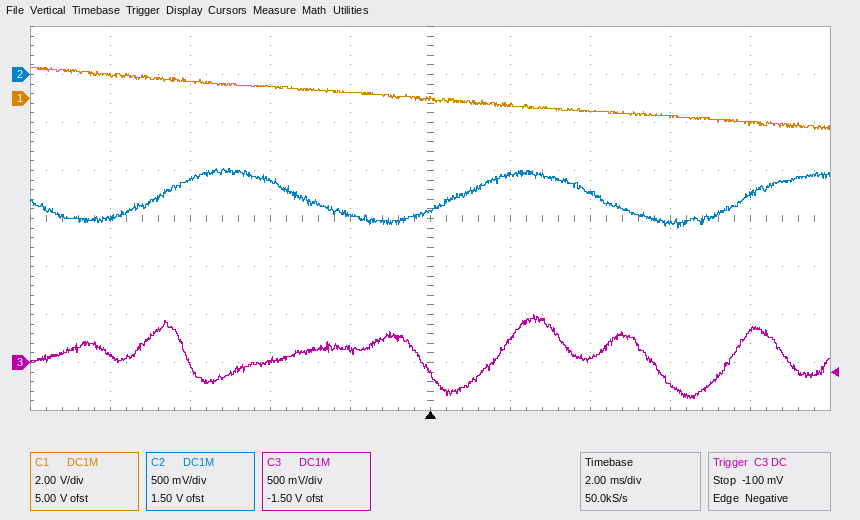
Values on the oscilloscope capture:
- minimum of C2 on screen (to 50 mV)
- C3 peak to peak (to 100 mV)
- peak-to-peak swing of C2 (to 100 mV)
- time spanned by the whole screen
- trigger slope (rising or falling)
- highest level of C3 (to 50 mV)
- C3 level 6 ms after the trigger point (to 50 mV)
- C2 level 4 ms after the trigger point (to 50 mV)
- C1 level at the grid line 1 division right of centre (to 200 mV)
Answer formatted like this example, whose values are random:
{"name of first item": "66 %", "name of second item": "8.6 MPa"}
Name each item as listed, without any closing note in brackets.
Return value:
{"minimum of C2 on screen": "-1.60 V", "C3 peak to peak": "900 mV", "peak-to-peak swing of C2": "600 mV", "time spanned by the whole screen": "20 ms", "trigger slope": "falling", "highest level of C3": "500 mV", "C3 level 6 ms after the trigger point": "-250 mV", "C2 level 4 ms after the trigger point": "-1.25 V", "C1 level at the grid line 1 division right of centre": "-200 mV"}
